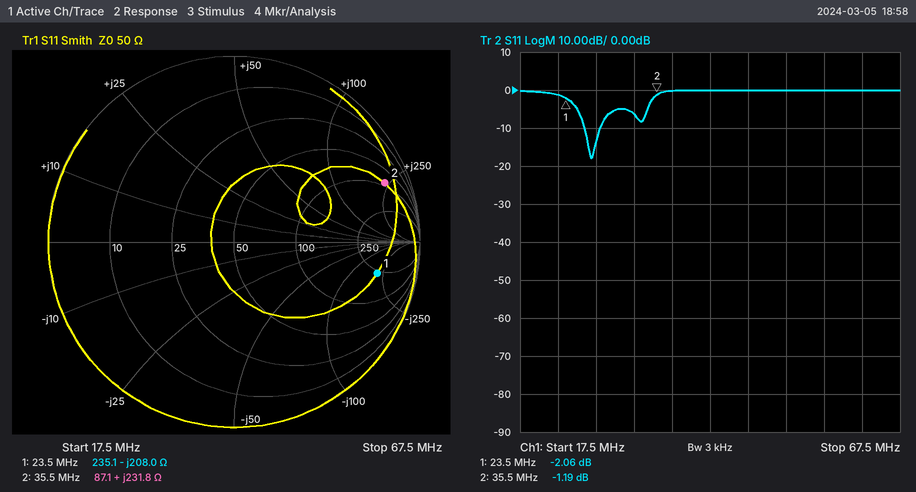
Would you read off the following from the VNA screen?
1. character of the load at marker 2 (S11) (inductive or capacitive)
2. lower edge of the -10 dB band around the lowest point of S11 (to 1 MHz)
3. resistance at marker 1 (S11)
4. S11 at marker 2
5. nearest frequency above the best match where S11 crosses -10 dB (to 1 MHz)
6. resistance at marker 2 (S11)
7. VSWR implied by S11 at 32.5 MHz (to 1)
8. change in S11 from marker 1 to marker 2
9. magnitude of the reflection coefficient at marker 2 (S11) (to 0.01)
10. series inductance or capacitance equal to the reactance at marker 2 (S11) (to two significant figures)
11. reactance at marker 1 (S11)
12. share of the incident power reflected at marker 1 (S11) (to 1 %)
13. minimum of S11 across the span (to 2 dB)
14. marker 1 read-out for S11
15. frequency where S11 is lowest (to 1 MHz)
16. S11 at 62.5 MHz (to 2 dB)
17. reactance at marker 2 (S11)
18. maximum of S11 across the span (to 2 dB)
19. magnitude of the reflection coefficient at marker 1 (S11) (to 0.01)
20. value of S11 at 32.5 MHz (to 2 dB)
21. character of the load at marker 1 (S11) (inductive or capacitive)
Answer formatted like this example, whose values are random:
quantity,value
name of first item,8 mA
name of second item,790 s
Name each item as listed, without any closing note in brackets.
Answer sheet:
quantity,value
character of the load at marker 2 (S11),inductive
lower edge of the -10 dB band around the lowest point of S11,26 MHz
resistance at marker 1,235.1 Ω
S11 at marker 2,-1.19 dB
nearest frequency above the best match where S11 crosses -10 dB,28 MHz
resistance at marker 2,87.1 Ω
VSWR implied by S11 at 32.5 MHz,3
change in S11 from marker 1 to marker 2,0.87 dB
magnitude of the reflection coefficient at marker 2 (S11),0.87
series inductance or capacitance equal to the reactance at marker 2 (S11),1.0 µH
reactance at marker 1,-208.0 Ω
share of the incident power reflected at marker 1 (S11),62 %
minimum of S11 across the span,-18 dB
marker 1 read-out for S11,-2.06 dB
frequency where S11 is lowest,27 MHz
S11 at 62.5 MHz,0 dB
reactance at marker 2,+231.8 Ω
maximum of S11 across the span,0 dB
magnitude of the reflection coefficient at marker 1 (S11),0.79
value of S11 at 32.5 MHz,-6 dB
character of the load at marker 1 (S11),capacitive
